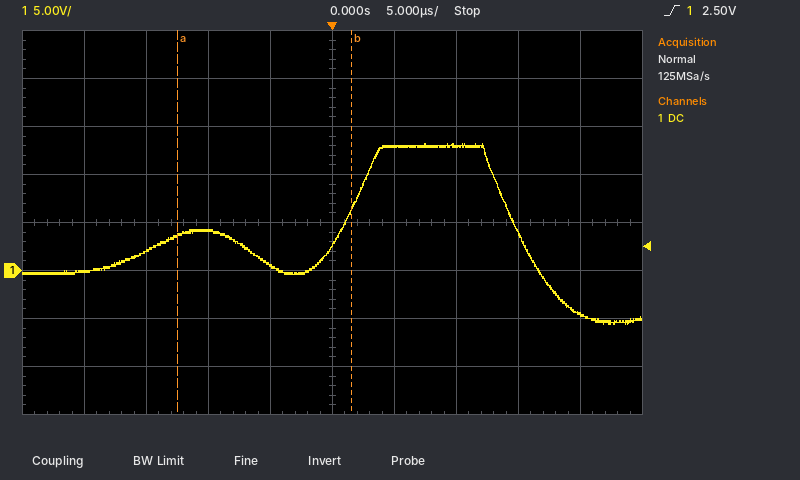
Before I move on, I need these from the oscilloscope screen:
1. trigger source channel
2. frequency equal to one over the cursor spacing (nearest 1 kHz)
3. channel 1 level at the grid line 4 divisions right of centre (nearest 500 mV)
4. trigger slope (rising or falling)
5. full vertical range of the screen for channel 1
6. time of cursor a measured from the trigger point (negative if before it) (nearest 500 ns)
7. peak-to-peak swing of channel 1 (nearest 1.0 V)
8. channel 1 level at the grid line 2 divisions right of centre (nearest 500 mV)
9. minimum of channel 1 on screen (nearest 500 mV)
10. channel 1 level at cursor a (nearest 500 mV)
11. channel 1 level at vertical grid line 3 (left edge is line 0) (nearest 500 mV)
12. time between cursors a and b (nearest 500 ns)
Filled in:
channel 1
71 kHz
-4.5 V
rising
40 V
-12.5 µs
19.0 V
13.0 V
-5.5 V
3.5 V
4.0 V
14.0 µs
